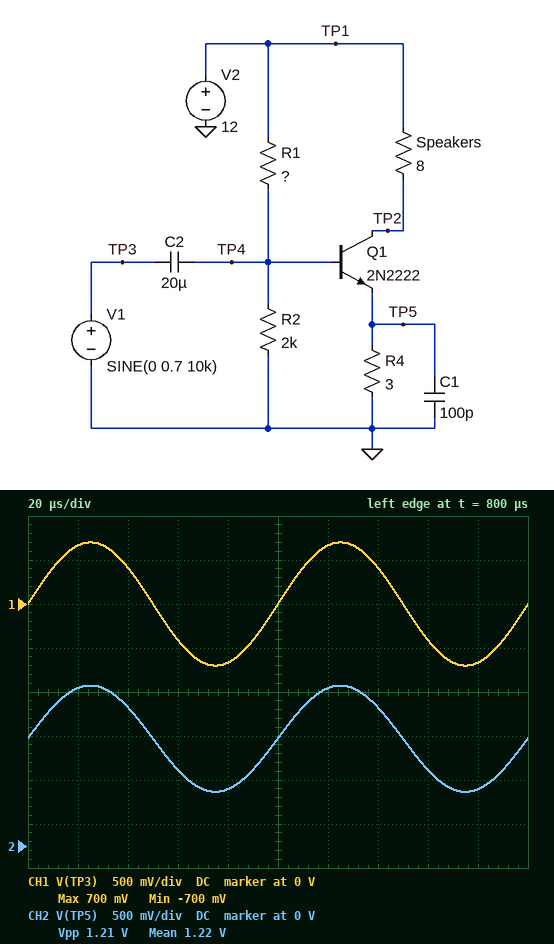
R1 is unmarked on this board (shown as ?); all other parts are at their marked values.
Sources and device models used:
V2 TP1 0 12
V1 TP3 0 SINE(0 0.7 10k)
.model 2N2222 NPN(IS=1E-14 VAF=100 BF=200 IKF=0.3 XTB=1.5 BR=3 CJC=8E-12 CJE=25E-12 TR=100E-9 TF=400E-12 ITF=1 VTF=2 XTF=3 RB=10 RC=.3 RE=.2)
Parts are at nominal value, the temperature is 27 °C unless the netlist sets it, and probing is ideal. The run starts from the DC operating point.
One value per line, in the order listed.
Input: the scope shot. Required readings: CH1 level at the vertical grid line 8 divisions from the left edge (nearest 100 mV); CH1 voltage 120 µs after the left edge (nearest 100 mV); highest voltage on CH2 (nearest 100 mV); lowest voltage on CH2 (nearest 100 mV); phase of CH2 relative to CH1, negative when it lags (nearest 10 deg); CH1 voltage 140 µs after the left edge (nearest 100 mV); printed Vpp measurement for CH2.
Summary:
-400 mV
700 mV
1.8 V
600 mV
0 deg
400 mV
1.21 V
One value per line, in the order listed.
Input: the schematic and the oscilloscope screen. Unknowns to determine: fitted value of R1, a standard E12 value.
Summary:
1.8 kΩ
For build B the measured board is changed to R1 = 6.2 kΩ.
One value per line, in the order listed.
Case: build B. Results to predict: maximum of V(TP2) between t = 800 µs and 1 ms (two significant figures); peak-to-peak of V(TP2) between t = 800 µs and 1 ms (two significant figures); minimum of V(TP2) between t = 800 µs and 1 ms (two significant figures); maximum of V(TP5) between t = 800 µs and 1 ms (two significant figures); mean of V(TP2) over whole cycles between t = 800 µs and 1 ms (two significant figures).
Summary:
12 V
2.8 V
9.2 V
1.1 V
11 V
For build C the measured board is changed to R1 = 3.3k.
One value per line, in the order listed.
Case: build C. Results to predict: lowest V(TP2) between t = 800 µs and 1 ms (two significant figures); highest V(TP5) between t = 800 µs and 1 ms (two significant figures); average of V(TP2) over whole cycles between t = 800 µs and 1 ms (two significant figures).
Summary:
8.3 V
1.4 V
9.9 V
